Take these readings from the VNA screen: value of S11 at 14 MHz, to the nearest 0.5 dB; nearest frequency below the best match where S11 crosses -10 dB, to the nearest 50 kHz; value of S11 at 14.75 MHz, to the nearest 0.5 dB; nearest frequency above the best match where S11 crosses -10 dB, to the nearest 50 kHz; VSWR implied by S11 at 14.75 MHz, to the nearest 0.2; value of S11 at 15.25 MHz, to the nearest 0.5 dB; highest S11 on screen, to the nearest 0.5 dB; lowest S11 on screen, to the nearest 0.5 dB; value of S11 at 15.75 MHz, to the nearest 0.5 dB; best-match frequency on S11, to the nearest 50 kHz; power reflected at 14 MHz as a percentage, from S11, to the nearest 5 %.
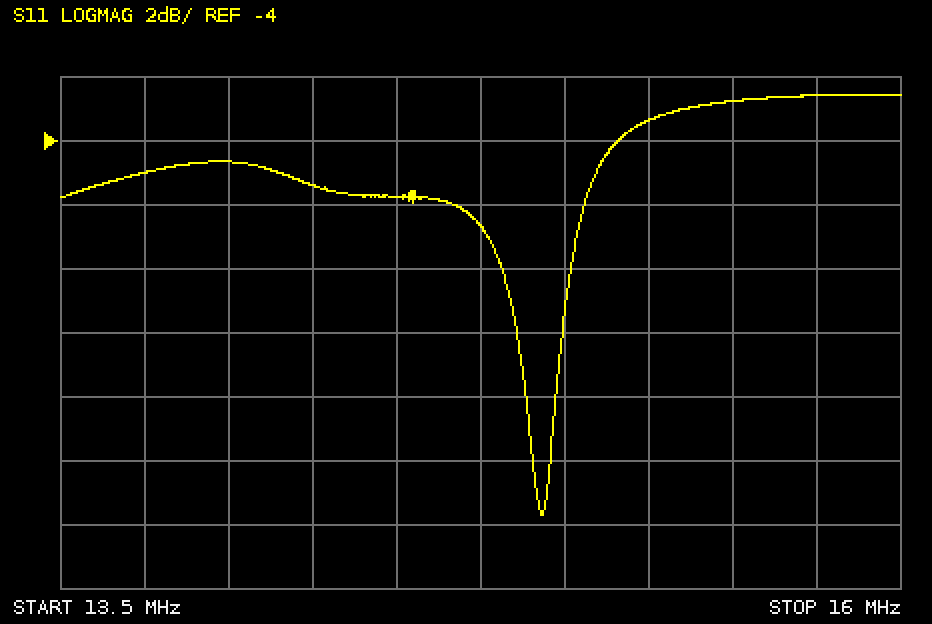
-4.5 dB
14.85 MHz
-6.5 dB
15.00 MHz
2.8
-3.5 dB
-2.5 dB
-15.5 dB
-2.5 dB
14.95 MHz
35 %
